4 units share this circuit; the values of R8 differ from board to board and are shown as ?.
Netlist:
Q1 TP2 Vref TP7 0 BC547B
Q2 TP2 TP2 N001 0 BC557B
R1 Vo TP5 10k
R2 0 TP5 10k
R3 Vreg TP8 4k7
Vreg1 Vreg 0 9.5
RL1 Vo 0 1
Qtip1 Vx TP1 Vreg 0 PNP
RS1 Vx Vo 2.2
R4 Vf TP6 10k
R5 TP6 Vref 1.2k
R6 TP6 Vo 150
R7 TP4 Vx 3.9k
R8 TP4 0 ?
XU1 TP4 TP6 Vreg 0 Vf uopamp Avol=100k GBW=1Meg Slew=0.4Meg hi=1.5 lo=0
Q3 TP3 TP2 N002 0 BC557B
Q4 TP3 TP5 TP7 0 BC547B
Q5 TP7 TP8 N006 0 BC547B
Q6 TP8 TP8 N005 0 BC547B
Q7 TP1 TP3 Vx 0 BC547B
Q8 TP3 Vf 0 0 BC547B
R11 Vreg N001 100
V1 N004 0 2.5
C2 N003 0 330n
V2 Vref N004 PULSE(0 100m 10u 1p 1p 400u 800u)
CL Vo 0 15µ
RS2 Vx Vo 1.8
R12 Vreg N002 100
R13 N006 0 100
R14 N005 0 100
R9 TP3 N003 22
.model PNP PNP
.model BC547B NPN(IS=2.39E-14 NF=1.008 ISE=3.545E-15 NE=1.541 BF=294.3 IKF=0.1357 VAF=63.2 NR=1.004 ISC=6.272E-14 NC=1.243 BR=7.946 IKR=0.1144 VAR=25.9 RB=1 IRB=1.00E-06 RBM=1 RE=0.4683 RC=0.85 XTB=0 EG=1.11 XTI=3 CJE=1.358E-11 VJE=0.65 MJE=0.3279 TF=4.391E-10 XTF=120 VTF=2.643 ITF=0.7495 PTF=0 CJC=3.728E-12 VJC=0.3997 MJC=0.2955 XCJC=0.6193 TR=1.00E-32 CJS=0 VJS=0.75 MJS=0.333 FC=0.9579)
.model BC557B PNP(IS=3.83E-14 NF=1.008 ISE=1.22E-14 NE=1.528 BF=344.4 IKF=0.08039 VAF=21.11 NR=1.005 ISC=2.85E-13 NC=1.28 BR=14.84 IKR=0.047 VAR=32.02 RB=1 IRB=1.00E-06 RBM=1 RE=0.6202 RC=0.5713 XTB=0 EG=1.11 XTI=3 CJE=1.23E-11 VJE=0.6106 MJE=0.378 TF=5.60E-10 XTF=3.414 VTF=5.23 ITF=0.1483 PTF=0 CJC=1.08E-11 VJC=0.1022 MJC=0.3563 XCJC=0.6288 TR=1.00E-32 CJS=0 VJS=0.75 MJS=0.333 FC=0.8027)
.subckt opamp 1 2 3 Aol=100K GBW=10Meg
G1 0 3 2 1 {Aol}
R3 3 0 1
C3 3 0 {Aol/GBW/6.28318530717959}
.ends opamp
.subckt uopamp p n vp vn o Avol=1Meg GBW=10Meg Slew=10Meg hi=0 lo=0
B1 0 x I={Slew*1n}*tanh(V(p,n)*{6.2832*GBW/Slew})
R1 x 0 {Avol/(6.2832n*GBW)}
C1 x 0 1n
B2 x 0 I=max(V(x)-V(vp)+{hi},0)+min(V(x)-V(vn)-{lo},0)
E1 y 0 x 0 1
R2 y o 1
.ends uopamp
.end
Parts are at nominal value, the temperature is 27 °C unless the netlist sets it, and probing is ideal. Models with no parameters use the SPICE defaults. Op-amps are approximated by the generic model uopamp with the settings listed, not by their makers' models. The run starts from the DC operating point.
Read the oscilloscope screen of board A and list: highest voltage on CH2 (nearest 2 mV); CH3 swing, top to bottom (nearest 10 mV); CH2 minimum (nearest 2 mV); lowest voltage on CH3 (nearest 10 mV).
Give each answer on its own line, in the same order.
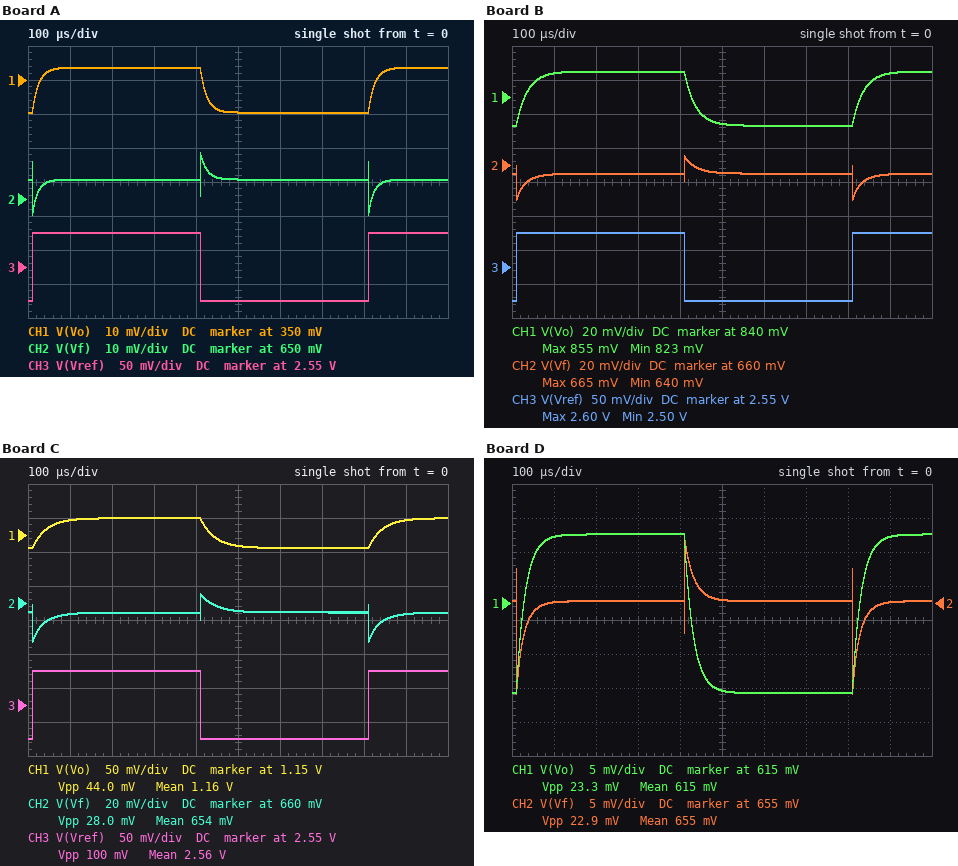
664 mV
100 mV
646 mV
2.50 V
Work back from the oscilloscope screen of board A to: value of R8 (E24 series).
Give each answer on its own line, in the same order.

24 kΩ
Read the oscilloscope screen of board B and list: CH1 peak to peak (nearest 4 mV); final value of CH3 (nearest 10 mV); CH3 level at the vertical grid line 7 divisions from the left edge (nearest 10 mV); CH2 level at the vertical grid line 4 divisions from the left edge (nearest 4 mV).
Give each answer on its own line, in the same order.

32 mV
2.60 V
2.50 V
656 mV
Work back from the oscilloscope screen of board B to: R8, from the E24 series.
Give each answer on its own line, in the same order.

6.2 kΩ
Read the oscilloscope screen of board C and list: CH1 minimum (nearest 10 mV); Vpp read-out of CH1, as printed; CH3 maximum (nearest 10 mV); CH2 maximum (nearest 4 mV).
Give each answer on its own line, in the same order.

1.13 V
44.0 mV
2.60 V
664 mV
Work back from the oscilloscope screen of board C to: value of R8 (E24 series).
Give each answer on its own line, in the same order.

5.1 kΩ
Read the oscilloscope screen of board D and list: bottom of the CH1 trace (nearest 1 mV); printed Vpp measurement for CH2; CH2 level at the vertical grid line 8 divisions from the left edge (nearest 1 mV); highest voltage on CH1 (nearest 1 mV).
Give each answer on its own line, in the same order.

602 mV
22.9 mV
655 mV
625 mV
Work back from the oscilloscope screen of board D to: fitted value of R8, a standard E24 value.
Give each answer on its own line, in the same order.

8.2 kΩ
